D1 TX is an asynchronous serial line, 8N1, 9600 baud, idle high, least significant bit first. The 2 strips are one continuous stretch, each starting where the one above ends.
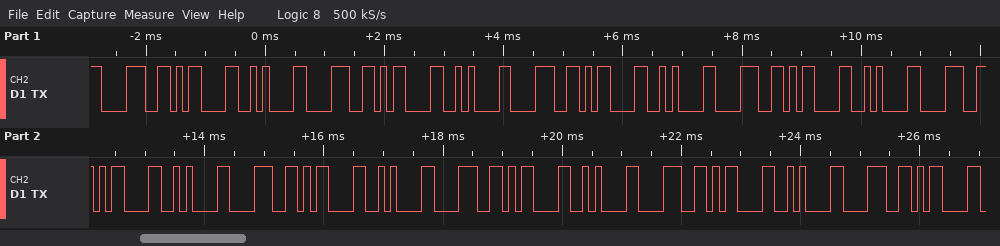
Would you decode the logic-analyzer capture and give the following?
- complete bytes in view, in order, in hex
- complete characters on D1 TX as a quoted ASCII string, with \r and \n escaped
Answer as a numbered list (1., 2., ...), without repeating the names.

1. 38 0D 0A 38 0D 0A 38 0D 0A 38 0D 0A 38 0D 0A 38 0D 0A 38 0D 0A 38 0D 0A 38 0D
2. "8\r\n8\r\n8\r\n8\r\n8\r\n8\r\n8\r\n8\r\n8\r"
